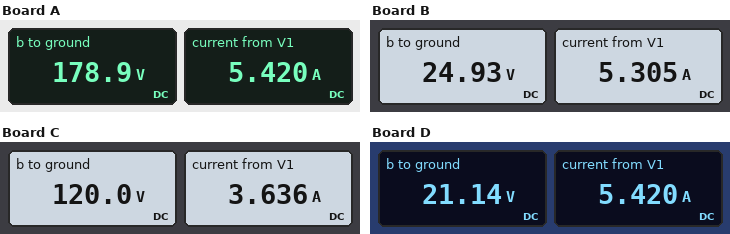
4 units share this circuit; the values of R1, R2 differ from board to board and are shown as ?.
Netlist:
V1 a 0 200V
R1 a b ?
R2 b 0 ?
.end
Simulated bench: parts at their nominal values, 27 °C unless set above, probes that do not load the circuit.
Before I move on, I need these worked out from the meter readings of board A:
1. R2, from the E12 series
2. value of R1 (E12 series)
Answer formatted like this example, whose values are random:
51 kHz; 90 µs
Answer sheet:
33 Ω; 3.9 Ω
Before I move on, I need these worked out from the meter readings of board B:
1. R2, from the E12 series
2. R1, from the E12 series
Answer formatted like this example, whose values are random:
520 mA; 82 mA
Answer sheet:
4.7 Ω; 33 Ω
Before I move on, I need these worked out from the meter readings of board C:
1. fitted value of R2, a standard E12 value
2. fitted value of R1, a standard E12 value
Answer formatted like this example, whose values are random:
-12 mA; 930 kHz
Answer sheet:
33 Ω; 22 Ω
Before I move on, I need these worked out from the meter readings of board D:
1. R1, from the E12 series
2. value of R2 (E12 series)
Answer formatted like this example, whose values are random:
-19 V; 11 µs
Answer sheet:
33 Ω; 3.9 Ω
